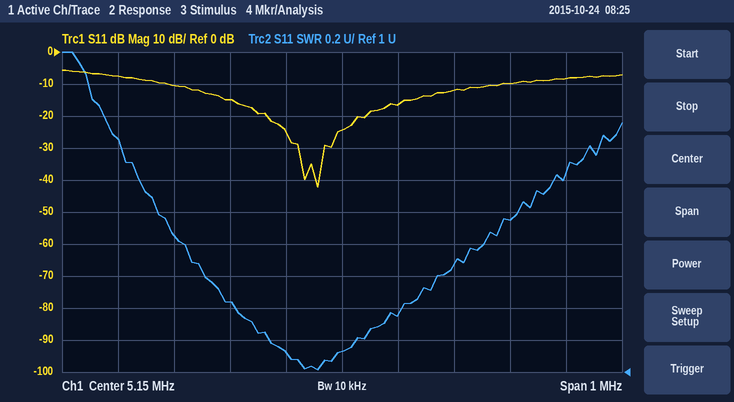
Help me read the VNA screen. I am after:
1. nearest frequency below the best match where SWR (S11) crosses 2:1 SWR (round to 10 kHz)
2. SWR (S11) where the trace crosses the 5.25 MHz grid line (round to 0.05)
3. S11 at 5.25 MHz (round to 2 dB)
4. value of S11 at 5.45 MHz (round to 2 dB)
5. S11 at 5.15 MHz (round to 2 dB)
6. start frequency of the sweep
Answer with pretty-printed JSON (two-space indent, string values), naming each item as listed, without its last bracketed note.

{
  "nearest frequency below the best match where SWR (S11) crosses 2:1 SWR": "4.82 MHz",
  "SWR (S11) where the trace crosses the 5.25 MHz grid line": "1.35",
  "S11 at 5.25 MHz": "-16 dB",
  "value of S11 at 5.45 MHz": "-10 dB",
  "S11 at 5.15 MHz": "-24 dB",
  "start frequency of the sweep": "4.65 MHz"
}
